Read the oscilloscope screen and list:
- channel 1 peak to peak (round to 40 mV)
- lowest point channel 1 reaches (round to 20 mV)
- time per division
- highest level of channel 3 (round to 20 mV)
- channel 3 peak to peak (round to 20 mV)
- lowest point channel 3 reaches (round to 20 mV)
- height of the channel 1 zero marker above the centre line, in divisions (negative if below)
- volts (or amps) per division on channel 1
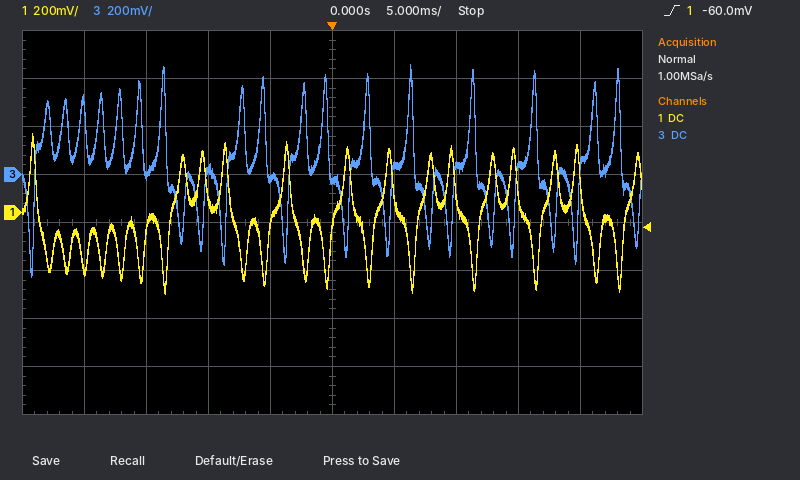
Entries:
680 mV
-340 mV
5 ms
460 mV
880 mV
-420 mV
+0.2 div
200 mV
